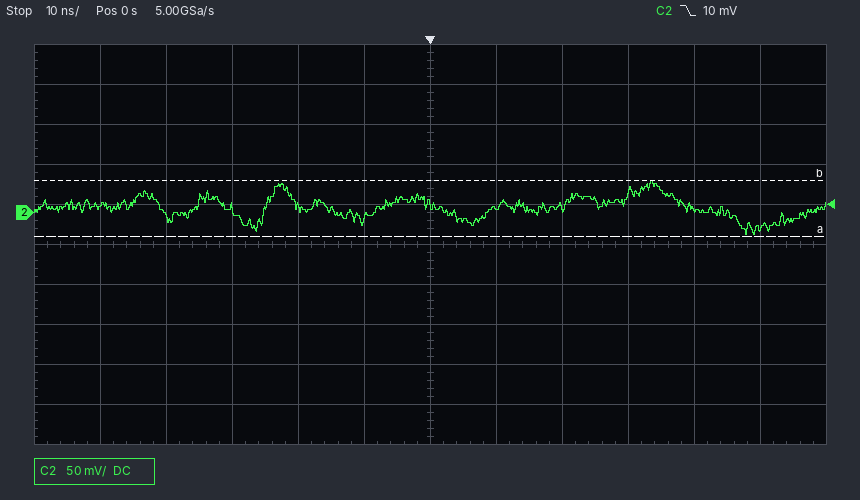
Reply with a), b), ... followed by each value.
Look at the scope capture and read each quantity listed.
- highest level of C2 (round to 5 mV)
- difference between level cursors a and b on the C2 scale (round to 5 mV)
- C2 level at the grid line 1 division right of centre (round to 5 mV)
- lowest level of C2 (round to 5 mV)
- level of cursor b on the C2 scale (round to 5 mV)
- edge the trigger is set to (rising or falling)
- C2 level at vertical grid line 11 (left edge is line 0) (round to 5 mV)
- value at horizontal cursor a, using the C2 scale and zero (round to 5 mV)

a) 40 mV
b) 70 mV
c) 5 mV
d) -30 mV
e) 40 mV
f) falling
g) -20 mV
h) -30 mV
